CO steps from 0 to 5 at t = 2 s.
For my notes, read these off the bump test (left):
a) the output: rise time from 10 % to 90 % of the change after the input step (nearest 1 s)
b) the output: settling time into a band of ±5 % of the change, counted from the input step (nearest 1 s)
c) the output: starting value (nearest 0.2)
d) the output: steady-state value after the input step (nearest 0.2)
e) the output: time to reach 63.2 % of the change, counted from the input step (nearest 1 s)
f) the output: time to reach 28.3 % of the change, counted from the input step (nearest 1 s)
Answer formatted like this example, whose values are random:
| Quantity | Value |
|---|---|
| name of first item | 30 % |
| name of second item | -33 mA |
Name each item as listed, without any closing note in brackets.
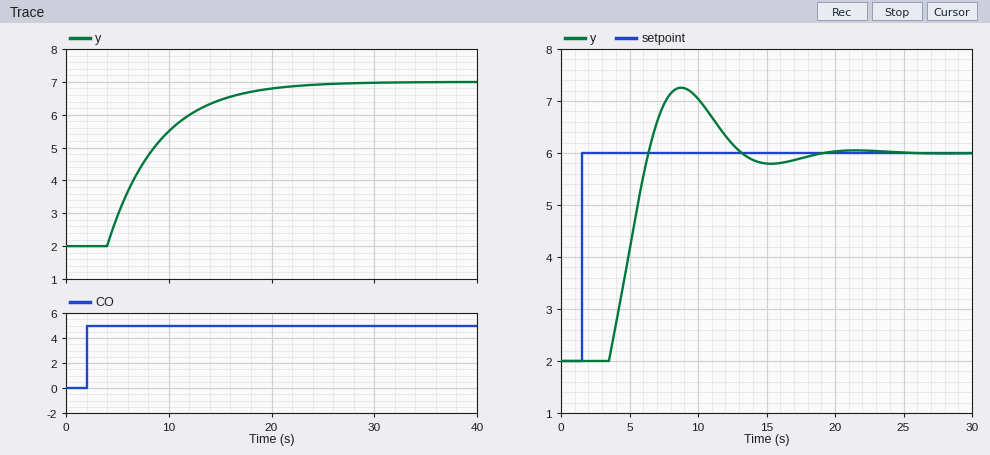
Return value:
| Quantity | Value |
|---|---|
| the output: rise time from 10 % to 90 % of the change after the input step | 11 s |
| the output: settling time into a band of ±5 % of the change, counted from the input step | 17 s |
| the output: starting value | 2.0 |
| the output: steady-state value after the input step | 7.0 |
| the output: time to reach 63.2 % of the change, counted from the input step | 7 s |
| the output: time to reach 28.3 % of the change, counted from the input step | 4 s |
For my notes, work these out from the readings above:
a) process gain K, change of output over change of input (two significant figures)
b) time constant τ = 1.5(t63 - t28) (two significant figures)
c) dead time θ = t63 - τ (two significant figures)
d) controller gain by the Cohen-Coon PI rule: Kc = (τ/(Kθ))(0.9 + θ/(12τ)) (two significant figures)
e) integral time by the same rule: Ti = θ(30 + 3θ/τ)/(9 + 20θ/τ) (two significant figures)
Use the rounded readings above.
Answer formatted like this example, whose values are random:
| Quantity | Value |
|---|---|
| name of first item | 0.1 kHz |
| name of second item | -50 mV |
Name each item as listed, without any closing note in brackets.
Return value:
| Quantity | Value |
|---|---|
| process gain K, change of output over change of input | 1.0 |
| time constant τ = 1.5(t63 - t28) | 4.5 s |
| dead time θ = t63 - τ | 2.5 s |
| controller gain by the Cohen-Coon PI rule: Kc = (τ/(Kθ))(0.9 + θ/(12τ)) | 1.7 |
| integral time by the same rule: Ti = θ(30 + 3θ/τ)/(9 + 20θ/τ) | 3.9 s |
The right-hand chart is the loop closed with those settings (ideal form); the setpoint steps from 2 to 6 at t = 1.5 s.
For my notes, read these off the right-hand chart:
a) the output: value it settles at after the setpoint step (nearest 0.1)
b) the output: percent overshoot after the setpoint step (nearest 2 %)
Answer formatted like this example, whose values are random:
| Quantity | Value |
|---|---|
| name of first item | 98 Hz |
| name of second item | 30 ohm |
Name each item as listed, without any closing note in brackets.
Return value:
| Quantity | Value |
|---|---|
| the output: value it settles at after the setpoint step | 6.0 |
| the output: percent overshoot after the setpoint step | 32 % |
